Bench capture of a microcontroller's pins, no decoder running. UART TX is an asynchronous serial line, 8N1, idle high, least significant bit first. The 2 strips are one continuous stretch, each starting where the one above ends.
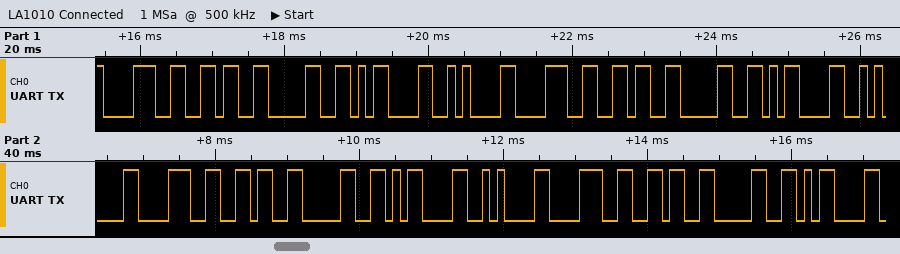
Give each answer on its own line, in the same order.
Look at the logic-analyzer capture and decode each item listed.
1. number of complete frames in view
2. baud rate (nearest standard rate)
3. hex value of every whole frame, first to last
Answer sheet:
19
9600 baud
0x38 0x36 0x30 0x0D 0x0A 0x38 0x36 0x30 0x0D 0x0A 0x38 0x36 0x30 0x0D 0x0A 0x38 0x36 0x30 0x0D
